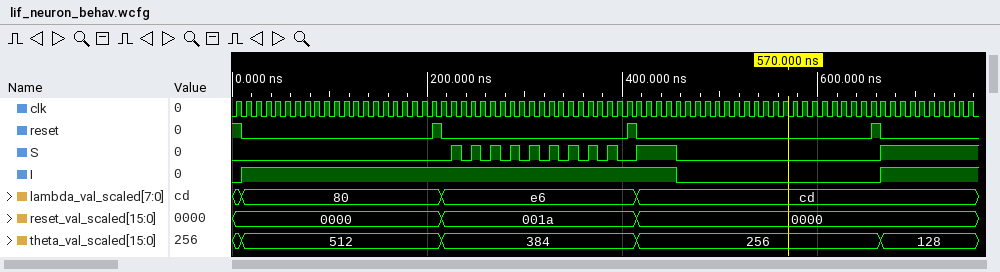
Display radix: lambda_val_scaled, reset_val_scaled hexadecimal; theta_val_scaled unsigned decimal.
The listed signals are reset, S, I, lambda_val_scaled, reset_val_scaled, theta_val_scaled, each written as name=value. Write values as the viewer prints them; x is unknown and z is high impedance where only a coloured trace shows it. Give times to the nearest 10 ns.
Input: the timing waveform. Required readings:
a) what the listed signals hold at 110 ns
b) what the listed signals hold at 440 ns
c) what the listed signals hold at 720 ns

reset=0, S=0, I=1, lambda_val_scaled=80, reset_val_scaled=0000, theta_val_scaled=512
reset=0, S=1, I=1, lambda_val_scaled=cd, reset_val_scaled=0000, theta_val_scaled=256
reset=0, S=1, I=1, lambda_val_scaled=cd, reset_val_scaled=0000, theta_val_scaled=128
